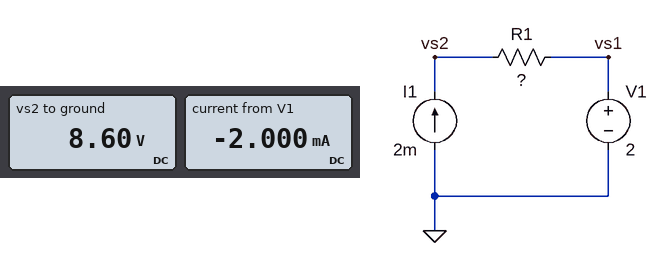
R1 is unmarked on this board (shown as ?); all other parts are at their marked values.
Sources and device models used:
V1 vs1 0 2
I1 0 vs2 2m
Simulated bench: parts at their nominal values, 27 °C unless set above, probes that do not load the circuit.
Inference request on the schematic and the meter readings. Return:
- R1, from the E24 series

3.3 kΩ
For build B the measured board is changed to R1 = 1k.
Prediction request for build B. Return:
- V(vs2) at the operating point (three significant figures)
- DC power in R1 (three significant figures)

4.00 V
4.00 mW
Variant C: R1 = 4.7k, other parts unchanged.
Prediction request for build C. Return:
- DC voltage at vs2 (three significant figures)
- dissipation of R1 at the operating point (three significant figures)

11.4 V
18.8 mW
